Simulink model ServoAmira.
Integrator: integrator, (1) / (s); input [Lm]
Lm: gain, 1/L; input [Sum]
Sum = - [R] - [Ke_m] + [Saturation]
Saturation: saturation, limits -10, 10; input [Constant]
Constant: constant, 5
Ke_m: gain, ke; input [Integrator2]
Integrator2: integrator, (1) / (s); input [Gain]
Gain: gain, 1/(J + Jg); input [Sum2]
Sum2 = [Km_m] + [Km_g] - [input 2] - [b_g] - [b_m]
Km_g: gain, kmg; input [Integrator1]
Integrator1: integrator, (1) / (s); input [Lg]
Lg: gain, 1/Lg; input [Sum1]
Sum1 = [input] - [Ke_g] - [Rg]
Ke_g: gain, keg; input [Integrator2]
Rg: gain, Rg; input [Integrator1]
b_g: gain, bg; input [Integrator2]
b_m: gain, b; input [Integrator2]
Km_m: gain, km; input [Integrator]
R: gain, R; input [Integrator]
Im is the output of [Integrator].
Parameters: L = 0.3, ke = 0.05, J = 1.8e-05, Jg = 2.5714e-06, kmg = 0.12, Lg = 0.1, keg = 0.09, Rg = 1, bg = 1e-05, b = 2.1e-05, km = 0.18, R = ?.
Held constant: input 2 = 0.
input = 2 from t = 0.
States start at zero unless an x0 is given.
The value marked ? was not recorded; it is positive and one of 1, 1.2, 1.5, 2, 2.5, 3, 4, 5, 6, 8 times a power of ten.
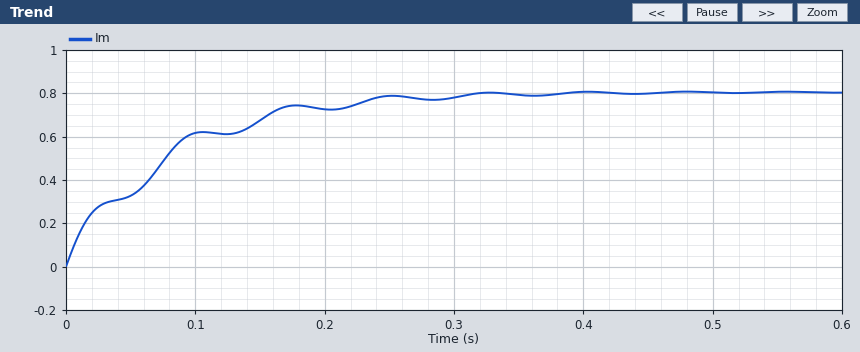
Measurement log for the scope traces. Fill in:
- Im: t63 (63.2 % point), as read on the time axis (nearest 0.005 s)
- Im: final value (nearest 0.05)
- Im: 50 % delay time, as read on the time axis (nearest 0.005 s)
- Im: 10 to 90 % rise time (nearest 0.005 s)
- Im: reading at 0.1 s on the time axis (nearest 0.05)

0.080 s
0.80
0.065 s
0.160 s
0.60
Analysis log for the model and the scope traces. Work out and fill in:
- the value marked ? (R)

4
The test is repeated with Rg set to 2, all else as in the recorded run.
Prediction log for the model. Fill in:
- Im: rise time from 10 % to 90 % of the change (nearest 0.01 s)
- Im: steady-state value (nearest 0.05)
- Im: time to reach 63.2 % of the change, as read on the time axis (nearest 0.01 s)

0.15 s
0.70
0.07 s
